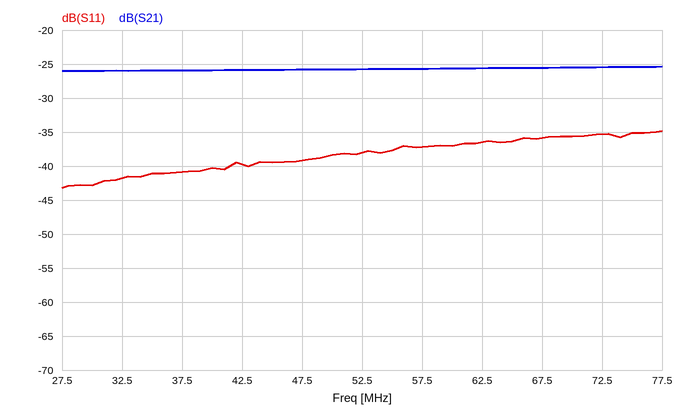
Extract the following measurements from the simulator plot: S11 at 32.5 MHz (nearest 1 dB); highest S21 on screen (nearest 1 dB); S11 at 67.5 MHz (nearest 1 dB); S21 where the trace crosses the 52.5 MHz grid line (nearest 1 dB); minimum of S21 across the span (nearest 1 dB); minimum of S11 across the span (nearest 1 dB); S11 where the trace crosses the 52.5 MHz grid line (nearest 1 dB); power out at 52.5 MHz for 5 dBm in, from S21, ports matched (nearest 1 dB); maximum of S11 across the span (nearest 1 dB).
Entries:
-42 dB
-25 dB
-36 dB
-26 dB
-26 dB
-43 dB
-38 dB
-21 dBm
-35 dB
